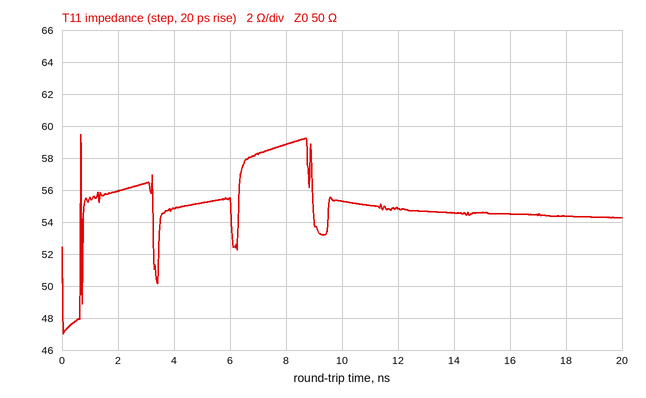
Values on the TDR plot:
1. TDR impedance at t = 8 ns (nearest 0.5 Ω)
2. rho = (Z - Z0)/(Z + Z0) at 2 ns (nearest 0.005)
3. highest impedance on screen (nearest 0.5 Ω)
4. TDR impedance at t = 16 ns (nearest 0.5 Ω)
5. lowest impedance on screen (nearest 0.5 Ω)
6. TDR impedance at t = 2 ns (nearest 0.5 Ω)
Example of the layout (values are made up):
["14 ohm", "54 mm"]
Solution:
["59.0 Ω", "+0.055", "59.5 Ω", "54.5 Ω", "47.0 Ω", "56.0 Ω"]
